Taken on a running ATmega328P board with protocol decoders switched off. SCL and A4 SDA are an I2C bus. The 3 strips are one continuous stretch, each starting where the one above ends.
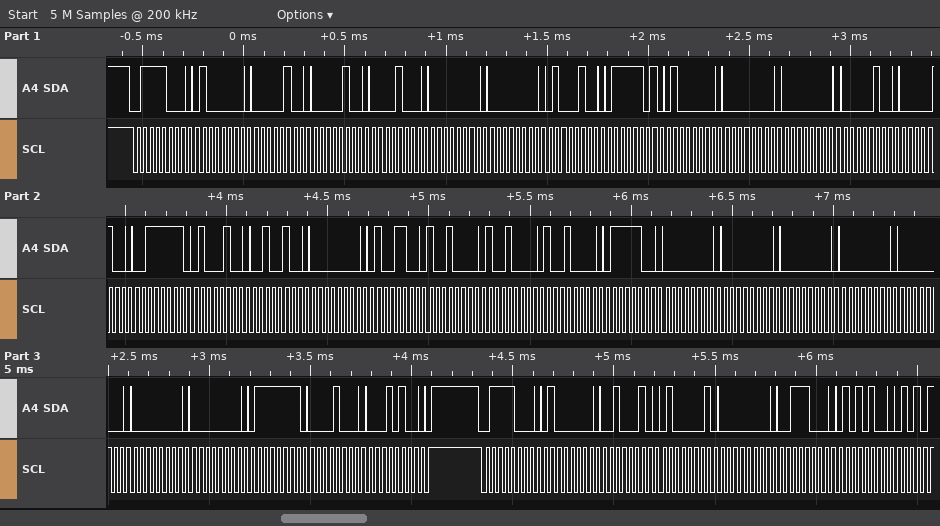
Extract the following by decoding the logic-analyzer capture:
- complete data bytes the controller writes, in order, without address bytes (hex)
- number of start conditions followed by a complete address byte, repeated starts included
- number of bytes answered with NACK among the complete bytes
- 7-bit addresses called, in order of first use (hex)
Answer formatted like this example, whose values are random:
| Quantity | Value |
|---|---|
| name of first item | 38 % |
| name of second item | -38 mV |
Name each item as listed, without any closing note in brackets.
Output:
| Quantity | Value |
|---|---|
| complete data bytes the controller writes, in order, without address bytes | 40 04 04 08 00 00 44 7D 40 00 00 04 04 3F 44 24 00 4C 90 90 90 7C 00 00 00 00 00 00 00 7F 08 14 40 22 41 00 38 54 |
| number of start conditions followed by a complete address byte, repeated starts included | 2 |
| number of bytes answered with NACK among the complete bytes | 0 |
| 7-bit addresses called, in order of first use | 0x3C |
